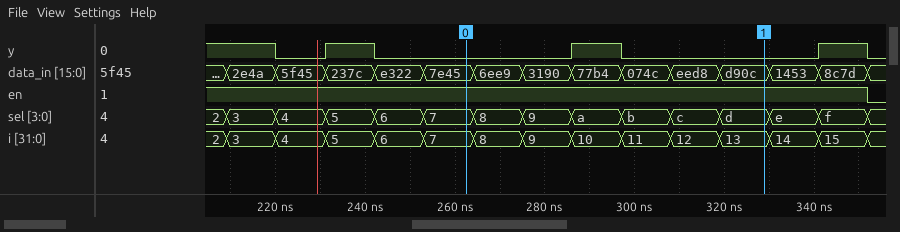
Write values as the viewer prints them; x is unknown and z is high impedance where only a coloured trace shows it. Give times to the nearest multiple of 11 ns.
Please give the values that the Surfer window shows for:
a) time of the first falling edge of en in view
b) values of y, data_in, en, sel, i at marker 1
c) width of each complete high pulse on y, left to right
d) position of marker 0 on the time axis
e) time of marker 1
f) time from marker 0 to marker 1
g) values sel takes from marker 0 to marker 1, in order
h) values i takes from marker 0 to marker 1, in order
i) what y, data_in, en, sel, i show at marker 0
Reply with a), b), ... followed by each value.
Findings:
a) 352 ns
b) y=0, data_in=d90c, en=1, sel=d, i=13
c) 11 ns, 11 ns, 11 ns
d) 264 ns
e) 330 ns
f) 66 ns
g) 7, 8, 9, a, b, c, d
h) 7, 8, 9, 10, 11, 12, 13
i) y=0, data_in=7e45, en=1, sel=7, i=7
